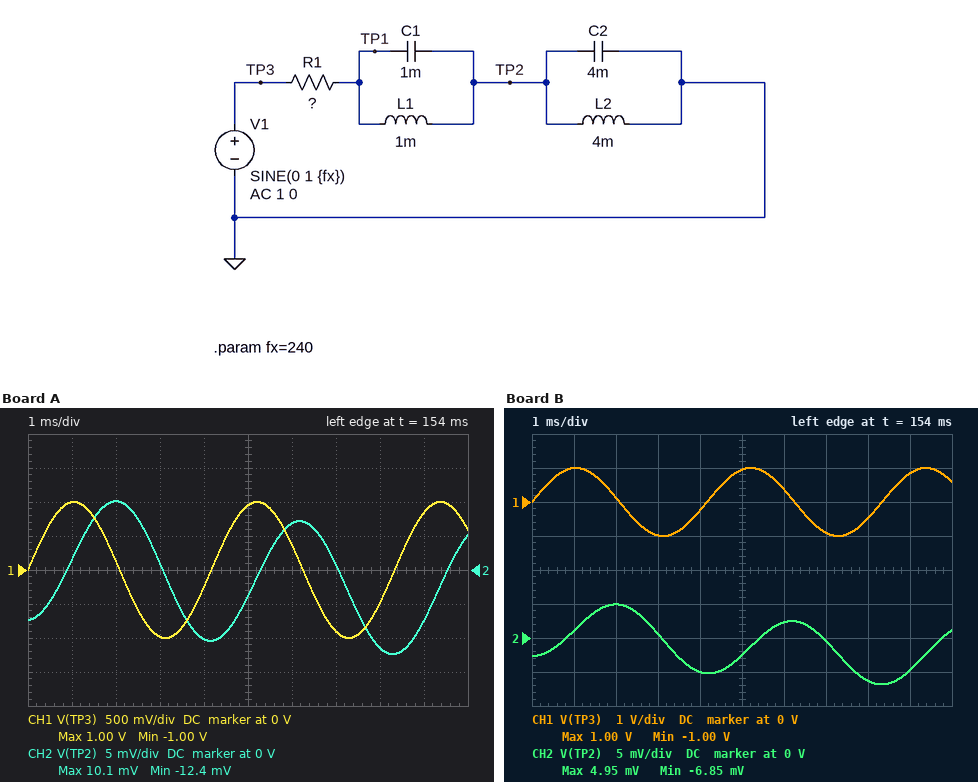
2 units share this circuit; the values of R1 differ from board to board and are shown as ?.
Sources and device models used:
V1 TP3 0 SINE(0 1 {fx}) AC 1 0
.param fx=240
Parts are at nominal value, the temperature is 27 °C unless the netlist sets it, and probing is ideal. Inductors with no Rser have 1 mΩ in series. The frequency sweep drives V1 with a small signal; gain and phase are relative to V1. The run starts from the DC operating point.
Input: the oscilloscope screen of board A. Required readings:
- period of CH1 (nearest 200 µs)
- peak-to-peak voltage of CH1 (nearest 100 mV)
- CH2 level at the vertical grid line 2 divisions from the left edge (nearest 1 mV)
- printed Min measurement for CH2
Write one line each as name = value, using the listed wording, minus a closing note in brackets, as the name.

period of CH1 = 4.2 ms
peak-to-peak voltage of CH1 = 2.0 V
CH2 level at the vertical grid line 2 divisions from the left edge = 10 mV
printed Min measurement for CH2 = -12.4 mV
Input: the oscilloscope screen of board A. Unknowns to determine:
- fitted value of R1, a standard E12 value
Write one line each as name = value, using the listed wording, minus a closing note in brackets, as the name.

fitted value of R1, a standard E12 value = 18 Ω
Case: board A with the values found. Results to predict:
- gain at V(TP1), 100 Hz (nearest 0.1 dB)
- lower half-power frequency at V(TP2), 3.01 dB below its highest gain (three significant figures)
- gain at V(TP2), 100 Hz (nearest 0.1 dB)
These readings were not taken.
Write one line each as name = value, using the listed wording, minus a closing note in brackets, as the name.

gain at V(TP1), 100 Hz = -30.1 dB
lower half-power frequency at V(TP2), 3.01 dB below its highest gain = 38.7 Hz
gain at V(TP2), 100 Hz = -31.6 dB
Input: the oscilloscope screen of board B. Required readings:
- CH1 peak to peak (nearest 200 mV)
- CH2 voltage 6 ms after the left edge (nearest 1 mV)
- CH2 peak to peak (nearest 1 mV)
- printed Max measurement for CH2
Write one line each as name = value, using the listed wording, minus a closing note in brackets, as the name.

CH1 peak to peak = 2.0 V
CH2 voltage 6 ms after the left edge = 2 mV
CH2 peak to peak = 12 mV
printed Max measurement for CH2 = 4.95 mV
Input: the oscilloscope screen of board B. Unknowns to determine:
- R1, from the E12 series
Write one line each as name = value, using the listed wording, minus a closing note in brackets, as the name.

R1, from the E12 series = 39 Ω
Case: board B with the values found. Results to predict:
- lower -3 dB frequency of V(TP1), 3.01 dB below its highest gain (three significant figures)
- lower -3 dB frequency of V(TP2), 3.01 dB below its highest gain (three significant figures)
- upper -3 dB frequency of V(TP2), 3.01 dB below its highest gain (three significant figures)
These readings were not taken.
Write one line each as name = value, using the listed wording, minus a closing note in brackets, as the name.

lower -3 dB frequency of V(TP1), 3.01 dB below its highest gain = 39.3 Hz
lower -3 dB frequency of V(TP2), 3.01 dB below its highest gain = 39.3 Hz
upper -3 dB frequency of V(TP2), 3.01 dB below its highest gain = 40.3 Hz
